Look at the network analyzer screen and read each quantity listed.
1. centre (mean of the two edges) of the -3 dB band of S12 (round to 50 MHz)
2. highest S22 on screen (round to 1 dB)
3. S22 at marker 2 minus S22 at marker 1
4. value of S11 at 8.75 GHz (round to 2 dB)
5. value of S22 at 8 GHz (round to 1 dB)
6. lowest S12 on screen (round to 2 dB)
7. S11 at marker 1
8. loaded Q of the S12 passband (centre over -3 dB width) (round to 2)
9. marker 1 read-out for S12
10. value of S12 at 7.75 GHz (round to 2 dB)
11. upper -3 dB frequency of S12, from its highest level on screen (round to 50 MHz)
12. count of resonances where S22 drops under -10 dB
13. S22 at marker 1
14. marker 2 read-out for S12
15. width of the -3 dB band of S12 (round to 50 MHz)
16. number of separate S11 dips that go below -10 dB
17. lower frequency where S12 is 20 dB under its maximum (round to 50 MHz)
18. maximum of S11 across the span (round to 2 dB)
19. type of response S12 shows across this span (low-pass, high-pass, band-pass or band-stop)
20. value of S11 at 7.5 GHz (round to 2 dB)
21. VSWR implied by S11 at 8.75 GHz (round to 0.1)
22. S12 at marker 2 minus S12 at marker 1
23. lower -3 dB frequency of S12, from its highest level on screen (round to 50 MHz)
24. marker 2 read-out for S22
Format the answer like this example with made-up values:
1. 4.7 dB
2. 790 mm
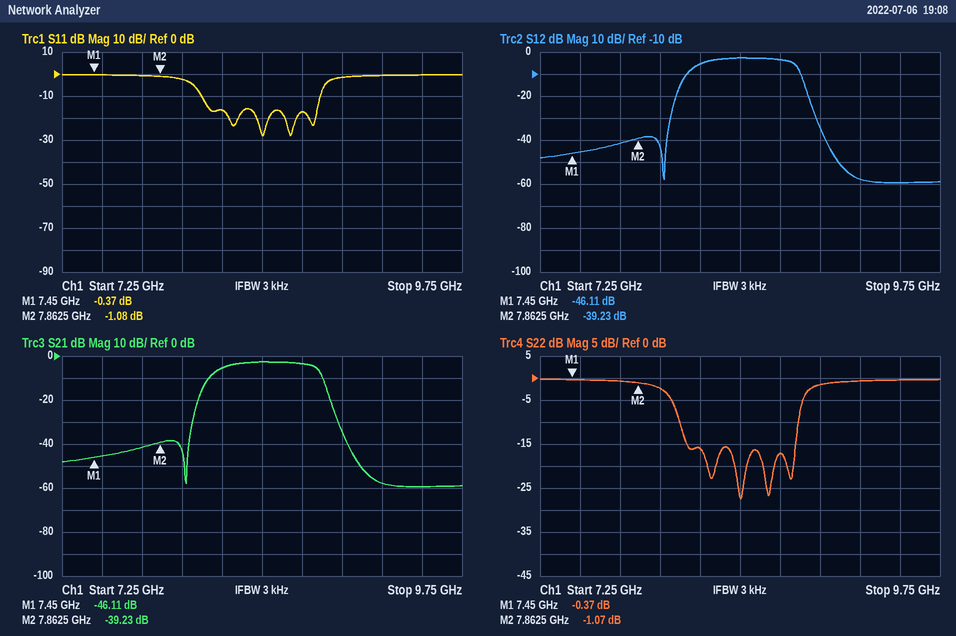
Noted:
1. 8.55 GHz
2. 0 dB
3. -0.70 dB
4. -18 dB
5. -2 dB
6. -60 dB
7. -0.37 dB
8. 14
9. -46.11 dB
10. -42 dB
11. 8.85 GHz
12. 4
13. -0.37 dB
14. -39.23 dB
15. 600 MHz
16. 4
17. 8.10 GHz
18. 0 dB
19. band-pass
20. 0 dB
21. 1.3
22. 6.88 dB
23. 8.25 GHz
24. -1.07 dB
